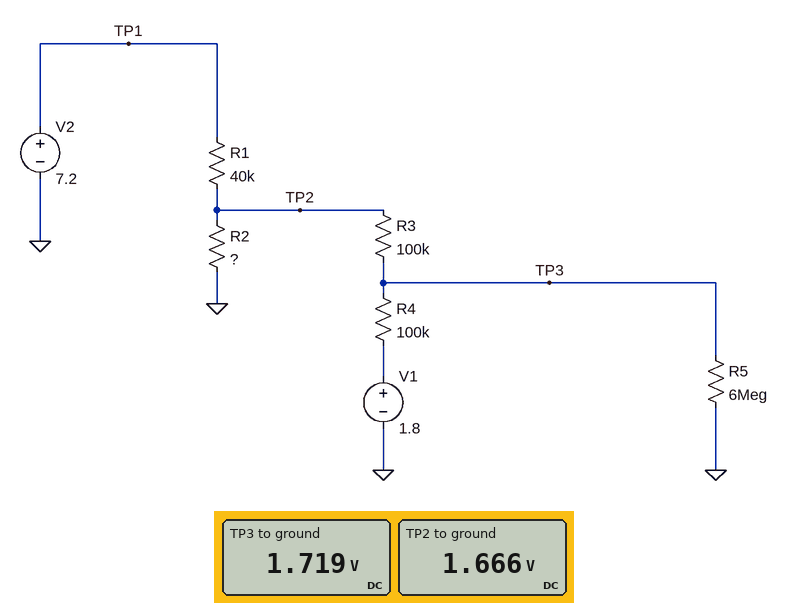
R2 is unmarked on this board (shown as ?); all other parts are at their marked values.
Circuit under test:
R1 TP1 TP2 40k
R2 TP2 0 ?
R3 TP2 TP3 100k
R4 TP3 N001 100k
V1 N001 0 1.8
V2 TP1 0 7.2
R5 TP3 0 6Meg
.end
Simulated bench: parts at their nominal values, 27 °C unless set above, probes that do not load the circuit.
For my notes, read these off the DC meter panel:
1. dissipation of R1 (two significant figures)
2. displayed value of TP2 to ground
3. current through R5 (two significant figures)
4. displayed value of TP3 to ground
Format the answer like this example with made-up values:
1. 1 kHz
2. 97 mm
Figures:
1. 770 µW
2. 1.666 V
3. 290 nA
4. 1.719 V
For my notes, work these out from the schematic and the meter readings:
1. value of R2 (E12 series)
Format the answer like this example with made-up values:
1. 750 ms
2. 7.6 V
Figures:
1. 12 kΩ
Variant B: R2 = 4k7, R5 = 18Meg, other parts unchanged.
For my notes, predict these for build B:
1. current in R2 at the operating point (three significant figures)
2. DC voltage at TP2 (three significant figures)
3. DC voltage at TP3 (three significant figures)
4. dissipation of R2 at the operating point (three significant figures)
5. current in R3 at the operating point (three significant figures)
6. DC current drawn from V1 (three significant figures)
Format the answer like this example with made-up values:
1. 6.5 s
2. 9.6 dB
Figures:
1. 166 µA
2. 778 mV
3. 1.29 V
4. 129 µW
5. 5.07 µA
6. 5.14 µA
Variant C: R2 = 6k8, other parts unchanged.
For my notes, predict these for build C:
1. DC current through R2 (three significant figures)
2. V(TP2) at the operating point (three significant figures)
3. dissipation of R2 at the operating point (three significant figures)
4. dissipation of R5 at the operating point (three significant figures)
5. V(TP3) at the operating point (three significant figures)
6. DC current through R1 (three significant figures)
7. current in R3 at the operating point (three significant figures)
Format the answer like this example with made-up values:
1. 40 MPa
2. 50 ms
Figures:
1. 157 µA
2. 1.07 V
3. 167 µW
4. 337 nW
5. 1.42 V
6. 153 µA
7. 3.55 µA
